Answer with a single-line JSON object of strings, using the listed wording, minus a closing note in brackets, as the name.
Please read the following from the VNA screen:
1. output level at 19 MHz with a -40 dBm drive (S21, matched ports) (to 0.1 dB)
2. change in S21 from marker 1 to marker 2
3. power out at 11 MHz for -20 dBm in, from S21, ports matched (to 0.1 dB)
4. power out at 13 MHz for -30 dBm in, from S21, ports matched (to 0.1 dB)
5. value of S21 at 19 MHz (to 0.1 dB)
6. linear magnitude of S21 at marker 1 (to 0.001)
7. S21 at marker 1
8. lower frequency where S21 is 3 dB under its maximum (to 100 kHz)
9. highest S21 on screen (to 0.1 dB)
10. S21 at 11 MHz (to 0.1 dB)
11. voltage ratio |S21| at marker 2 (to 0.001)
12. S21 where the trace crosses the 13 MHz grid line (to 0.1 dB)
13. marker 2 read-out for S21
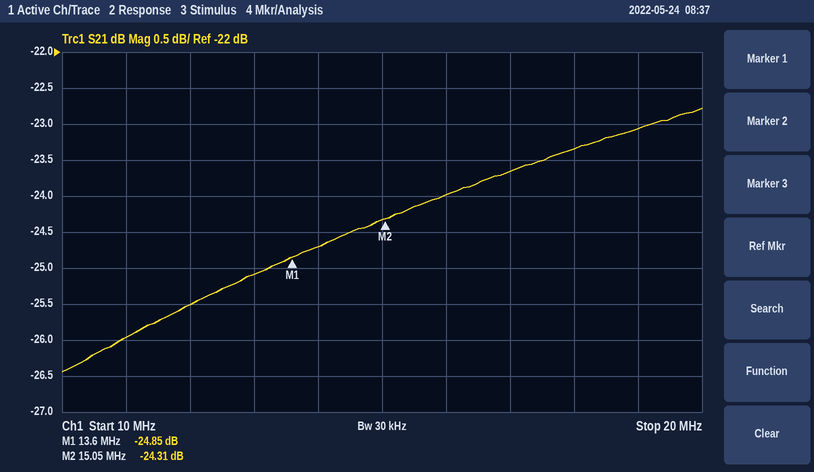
{"output level at 19 MHz with a -40 dBm drive (S21, matched ports)": "-63.1 dBm", "change in S21 from marker 1 to marker 2": "0.54 dB", "power out at 11 MHz for -20 dBm in, from S21, ports matched": "-46.0 dBm", "power out at 13 MHz for -30 dBm in, from S21, ports matched": "-55.1 dBm", "value of S21 at 19 MHz": "-23.1 dB", "linear magnitude of S21 at marker 1": "0.057", "S21 at marker 1": "-24.85 dB", "lower frequency where S21 is 3 dB under its maximum": "11.4 MHz", "highest S21 on screen": "-22.8 dB", "S21 at 11 MHz": "-26.0 dB", "voltage ratio |S21| at marker 2": "0.061", "S21 where the trace crosses the 13 MHz grid line": "-25.1 dB", "marker 2 read-out for S21": "-24.31 dB"}
